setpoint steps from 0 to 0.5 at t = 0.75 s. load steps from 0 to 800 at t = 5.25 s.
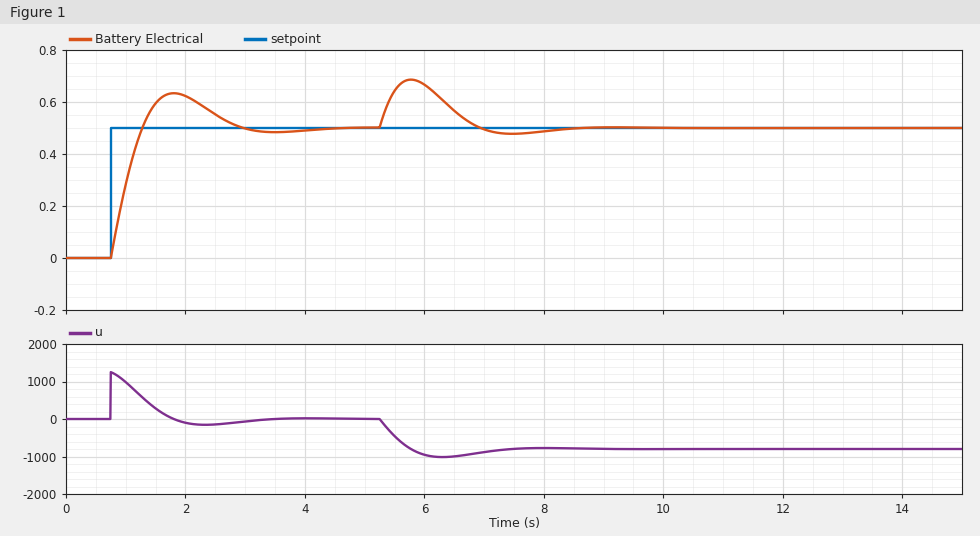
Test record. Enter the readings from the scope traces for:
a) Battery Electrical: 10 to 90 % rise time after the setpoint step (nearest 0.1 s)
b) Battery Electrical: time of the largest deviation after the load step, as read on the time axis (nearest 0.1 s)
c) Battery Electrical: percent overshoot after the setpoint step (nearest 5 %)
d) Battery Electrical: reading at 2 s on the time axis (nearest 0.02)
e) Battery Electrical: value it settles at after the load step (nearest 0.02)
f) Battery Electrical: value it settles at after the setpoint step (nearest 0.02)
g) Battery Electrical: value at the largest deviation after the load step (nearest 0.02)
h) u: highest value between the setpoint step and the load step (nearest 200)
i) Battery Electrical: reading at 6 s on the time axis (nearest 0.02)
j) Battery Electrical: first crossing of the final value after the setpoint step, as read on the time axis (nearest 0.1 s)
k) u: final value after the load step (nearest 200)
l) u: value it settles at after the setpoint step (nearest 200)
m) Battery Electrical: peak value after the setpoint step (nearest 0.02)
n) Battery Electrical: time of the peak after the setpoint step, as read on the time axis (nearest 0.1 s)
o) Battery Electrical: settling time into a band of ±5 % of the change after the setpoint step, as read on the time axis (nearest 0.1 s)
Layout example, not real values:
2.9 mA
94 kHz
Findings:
0.4 s
5.8 s
25 %
0.62
0.50
0.50
0.68
1200
0.66
1.3 s
-800
0
0.64
1.8 s
2.7 s
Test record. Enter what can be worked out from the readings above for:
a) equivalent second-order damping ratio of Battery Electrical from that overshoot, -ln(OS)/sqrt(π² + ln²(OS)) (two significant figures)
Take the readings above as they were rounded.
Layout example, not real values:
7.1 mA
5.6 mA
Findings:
0.40
